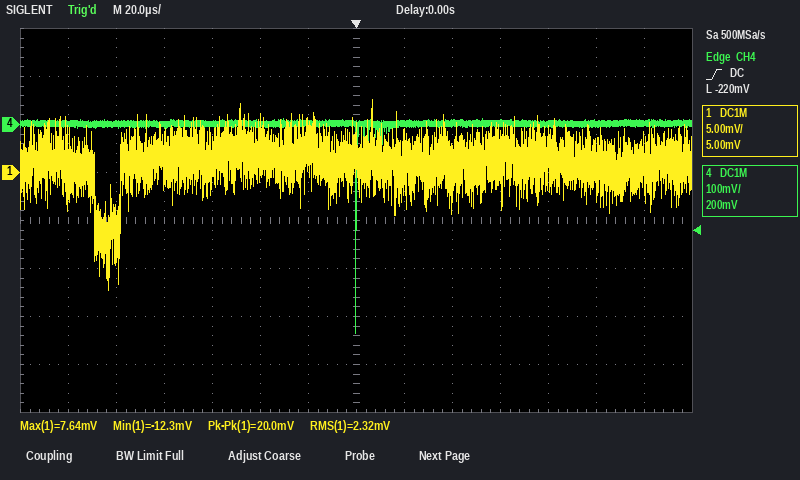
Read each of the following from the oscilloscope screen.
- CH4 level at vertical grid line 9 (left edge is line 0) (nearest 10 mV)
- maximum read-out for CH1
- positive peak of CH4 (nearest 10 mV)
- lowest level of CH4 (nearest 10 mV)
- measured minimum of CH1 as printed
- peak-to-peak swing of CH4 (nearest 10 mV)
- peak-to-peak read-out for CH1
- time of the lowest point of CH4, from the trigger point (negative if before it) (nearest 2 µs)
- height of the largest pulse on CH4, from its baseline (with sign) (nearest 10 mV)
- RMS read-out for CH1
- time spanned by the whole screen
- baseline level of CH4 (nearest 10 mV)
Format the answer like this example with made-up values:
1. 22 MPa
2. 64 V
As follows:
1. 0 mV
2. 7.64 mV
3. 10 mV
4. -440 mV
5. -12.3 mV
6. 450 mV
7. 20.0 mV
8. 0 µs
9. -440 mV
10. 2.32 mV
11. 280 µs
12. 0 mV
